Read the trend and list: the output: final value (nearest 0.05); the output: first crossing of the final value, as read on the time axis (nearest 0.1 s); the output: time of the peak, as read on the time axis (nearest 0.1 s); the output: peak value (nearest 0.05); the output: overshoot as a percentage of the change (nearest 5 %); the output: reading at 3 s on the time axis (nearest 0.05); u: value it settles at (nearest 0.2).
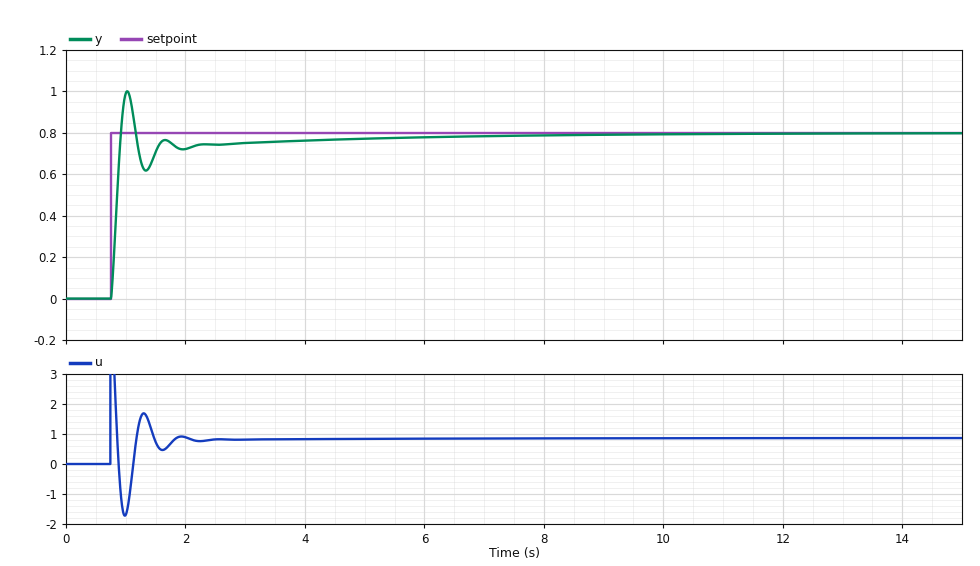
0.80
0.9 s
1.0 s
1.00
25 %
0.75
0.8
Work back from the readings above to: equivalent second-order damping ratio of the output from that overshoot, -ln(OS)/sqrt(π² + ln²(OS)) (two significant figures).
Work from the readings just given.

0.40
